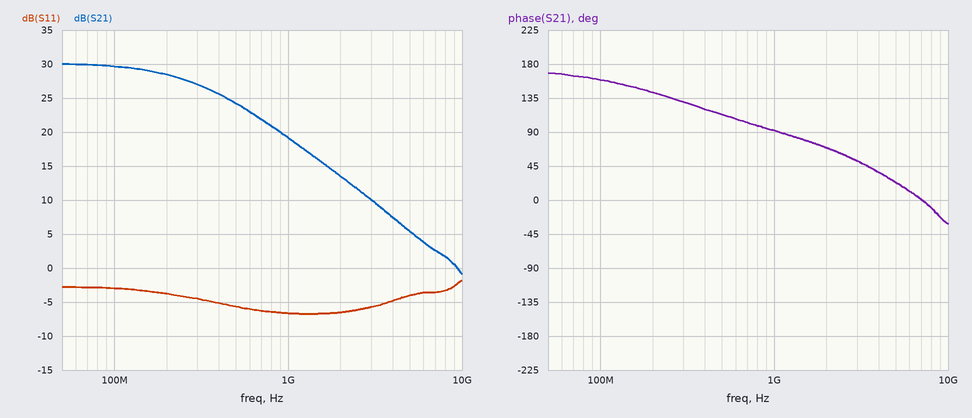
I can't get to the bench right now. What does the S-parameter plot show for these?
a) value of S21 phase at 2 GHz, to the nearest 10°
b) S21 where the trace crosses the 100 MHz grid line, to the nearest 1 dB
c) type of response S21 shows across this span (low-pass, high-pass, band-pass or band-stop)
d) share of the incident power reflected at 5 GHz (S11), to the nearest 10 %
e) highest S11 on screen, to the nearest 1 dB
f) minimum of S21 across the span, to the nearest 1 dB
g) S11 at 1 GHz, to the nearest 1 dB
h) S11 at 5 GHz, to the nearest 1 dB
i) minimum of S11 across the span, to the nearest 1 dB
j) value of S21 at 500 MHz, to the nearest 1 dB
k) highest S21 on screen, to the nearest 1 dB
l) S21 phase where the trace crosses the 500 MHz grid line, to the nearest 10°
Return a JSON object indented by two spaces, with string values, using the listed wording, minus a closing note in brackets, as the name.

{
  "value of S21 phase at 2 GHz, to the nearest 10°": "70°",
  "S21 where the trace crosses the 100 MHz grid line, to the nearest 1 dB": "30 dB",
  "type of response S21 shows across this span": "low-pass",
  "share of the incident power reflected at 5 GHz (S11), to the nearest 10 %": "40 %",
  "highest S11 on screen, to the nearest 1 dB": "-2 dB",
  "minimum of S21 across the span, to the nearest 1 dB": "-1 dB",
  "S11 at 1 GHz, to the nearest 1 dB": "-7 dB",
  "S11 at 5 GHz, to the nearest 1 dB": "-4 dB",
  "minimum of S11 across the span, to the nearest 1 dB": "-7 dB",
  "value of S21 at 500 MHz, to the nearest 1 dB": "24 dB",
  "highest S21 on screen, to the nearest 1 dB": "30 dB",
  "S21 phase where the trace crosses the 500 MHz grid line, to the nearest 10°": "110°"
}
